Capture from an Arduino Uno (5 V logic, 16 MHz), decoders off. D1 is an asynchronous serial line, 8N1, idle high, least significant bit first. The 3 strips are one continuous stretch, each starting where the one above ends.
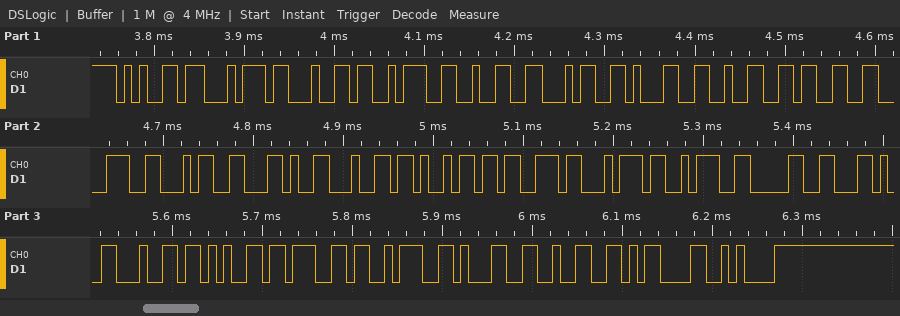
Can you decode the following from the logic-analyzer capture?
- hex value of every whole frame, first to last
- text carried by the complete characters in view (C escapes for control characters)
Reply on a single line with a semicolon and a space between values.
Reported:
0x65 0x74 0x64 0x3A 0x32 0x34 0x31 0x32 0x33 0x38 0x34 0x2C 0x64 0x69 0x73 0x74 0x3A 0x30 0x2C 0x64 0x65 0x67 0x3A 0x31 0x32 0x0D 0x0A; "etd:2412384,dist:0,deg:12\r\n"
